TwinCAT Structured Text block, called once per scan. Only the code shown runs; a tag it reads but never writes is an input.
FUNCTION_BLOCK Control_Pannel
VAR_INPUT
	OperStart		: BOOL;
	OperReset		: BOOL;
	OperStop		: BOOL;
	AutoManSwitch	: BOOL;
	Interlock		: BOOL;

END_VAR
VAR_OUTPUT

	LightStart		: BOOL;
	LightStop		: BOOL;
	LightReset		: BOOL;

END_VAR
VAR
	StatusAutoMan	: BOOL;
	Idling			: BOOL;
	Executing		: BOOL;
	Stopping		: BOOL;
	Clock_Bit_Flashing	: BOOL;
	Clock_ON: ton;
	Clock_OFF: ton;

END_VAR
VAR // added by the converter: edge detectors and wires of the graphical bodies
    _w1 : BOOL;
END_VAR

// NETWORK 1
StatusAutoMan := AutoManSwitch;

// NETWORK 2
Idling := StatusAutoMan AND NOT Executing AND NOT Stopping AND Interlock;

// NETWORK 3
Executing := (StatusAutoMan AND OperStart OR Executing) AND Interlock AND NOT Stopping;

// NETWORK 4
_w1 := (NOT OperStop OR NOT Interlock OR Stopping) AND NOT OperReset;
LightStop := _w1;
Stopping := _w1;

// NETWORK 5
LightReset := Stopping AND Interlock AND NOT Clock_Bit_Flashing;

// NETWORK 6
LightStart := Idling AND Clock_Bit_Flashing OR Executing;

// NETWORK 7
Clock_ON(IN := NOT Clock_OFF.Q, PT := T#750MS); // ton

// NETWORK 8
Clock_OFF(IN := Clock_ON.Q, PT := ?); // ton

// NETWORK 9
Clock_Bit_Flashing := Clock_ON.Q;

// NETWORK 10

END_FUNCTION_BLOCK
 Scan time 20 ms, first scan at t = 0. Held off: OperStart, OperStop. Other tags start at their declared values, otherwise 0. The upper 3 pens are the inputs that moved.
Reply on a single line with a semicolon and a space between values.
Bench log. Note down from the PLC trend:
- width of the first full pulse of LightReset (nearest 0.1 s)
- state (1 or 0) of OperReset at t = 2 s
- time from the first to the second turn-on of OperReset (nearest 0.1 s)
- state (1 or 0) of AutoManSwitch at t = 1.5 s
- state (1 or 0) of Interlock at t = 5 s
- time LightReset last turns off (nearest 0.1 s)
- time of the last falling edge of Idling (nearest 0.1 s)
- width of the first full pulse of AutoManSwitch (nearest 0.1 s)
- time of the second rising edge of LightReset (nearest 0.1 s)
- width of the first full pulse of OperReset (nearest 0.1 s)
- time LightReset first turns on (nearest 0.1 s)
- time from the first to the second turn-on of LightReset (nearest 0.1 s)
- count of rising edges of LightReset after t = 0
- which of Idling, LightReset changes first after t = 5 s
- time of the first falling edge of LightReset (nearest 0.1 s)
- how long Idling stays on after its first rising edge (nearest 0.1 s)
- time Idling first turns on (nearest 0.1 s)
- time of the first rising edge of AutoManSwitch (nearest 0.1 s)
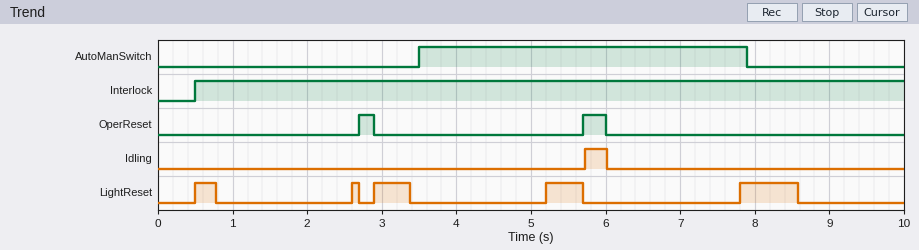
0.3 s; 0; 3.0 s; 0; 1; 8.6 s; 6.0 s; 4.4 s; 2.6 s; 0.2 s; 0.5 s; 2.1 s; 5; LightReset; 0.8 s; 0.3 s; 5.7 s; 3.5 s
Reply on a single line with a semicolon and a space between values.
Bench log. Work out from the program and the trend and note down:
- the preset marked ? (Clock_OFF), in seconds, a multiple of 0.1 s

1.8 s
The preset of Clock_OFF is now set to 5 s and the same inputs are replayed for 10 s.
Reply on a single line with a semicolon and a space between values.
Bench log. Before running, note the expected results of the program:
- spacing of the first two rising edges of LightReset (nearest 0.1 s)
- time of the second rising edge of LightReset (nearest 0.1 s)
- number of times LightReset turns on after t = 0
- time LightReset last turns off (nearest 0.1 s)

5.5 s; 6.0 s; 2; 6.6 s
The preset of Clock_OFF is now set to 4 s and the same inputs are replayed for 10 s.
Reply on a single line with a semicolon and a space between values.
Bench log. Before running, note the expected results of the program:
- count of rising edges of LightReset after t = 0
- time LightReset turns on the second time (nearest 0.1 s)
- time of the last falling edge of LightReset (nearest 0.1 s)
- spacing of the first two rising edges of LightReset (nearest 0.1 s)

3; 4.8 s; 5.6 s; 4.3 s
